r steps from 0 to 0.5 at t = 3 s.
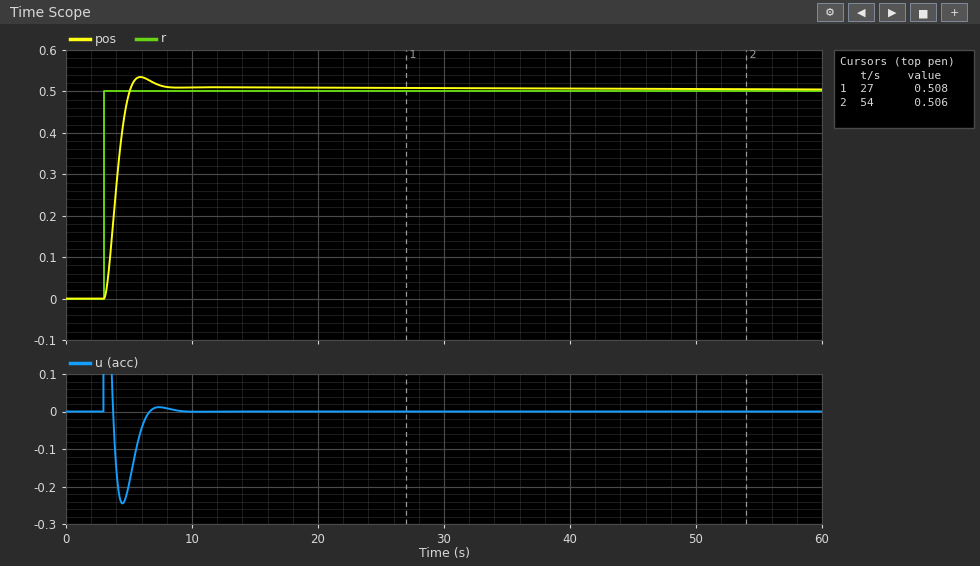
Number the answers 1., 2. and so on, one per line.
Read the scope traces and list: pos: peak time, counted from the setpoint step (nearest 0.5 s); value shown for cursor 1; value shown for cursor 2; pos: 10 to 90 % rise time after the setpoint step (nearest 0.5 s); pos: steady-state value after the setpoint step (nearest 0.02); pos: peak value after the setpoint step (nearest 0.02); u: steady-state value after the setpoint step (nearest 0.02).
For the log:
1. 3.0 s
2. 0.508
3. 0.506
4. 1.5 s
5. 0.50
6. 0.54
7. 0.00
